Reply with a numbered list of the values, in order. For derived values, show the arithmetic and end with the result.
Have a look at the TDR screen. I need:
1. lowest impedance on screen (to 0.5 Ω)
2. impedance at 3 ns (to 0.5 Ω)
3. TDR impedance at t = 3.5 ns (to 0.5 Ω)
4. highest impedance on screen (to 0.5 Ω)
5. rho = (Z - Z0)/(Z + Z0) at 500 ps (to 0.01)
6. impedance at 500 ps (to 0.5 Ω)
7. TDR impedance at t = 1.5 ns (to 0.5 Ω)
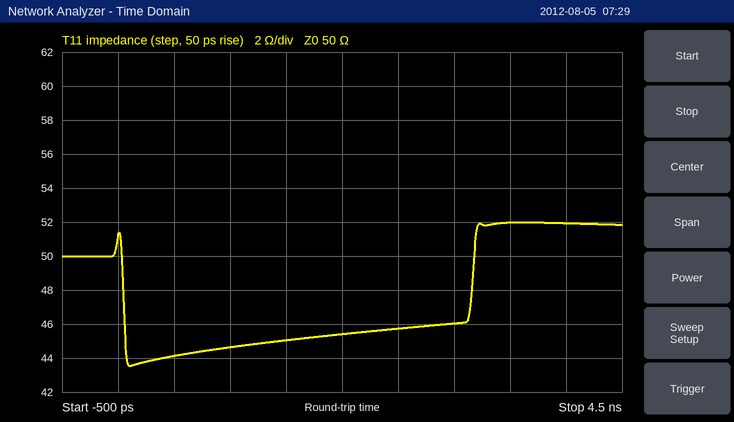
1. 43.5 Ω
2. 46.0 Ω
3. 52.0 Ω
4. 52.0 Ω
5. (44 − 50)/(44 + 50) ≈ -0.06
6. 44.0 Ω
7. 45.0 Ω
